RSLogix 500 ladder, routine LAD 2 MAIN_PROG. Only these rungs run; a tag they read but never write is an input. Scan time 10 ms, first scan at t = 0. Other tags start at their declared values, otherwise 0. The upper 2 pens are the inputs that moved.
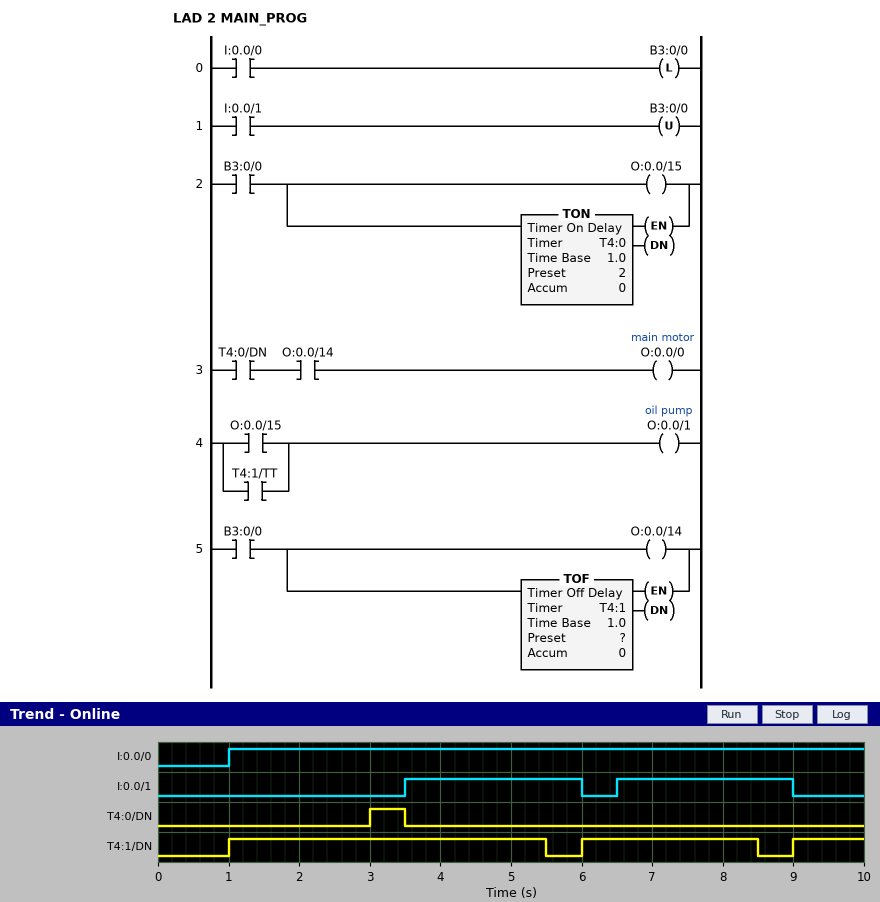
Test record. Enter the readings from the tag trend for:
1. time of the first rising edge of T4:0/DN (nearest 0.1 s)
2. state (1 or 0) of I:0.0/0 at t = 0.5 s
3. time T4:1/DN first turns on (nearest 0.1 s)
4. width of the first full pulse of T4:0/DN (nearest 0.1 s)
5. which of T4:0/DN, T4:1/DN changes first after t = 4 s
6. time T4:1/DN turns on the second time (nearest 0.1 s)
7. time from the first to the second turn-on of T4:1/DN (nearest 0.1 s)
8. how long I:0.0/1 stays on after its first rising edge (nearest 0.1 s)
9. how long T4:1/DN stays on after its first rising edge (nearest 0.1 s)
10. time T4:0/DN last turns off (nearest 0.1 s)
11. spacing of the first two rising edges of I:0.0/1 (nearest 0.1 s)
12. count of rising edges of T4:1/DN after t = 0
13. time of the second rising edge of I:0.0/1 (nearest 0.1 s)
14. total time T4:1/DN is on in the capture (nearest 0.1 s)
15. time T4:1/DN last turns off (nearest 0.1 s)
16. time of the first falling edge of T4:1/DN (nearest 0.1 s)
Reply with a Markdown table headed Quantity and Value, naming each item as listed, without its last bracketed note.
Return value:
| Quantity | Value |
|---|---|
| time of the first rising edge of T4:0/DN | 3.0 s |
| state (1 or 0) of I:0.0/0 at t = 0.5 s | 0 |
| time T4:1/DN first turns on | 1.0 s |
| width of the first full pulse of T4:0/DN | 0.5 s |
| which of T4:0/DN, T4:1/DN changes first after t = 4 s | T4:1/DN |
| time T4:1/DN turns on the second time | 6.0 s |
| time from the first to the second turn-on of T4:1/DN | 5.0 s |
| how long I:0.0/1 stays on after its first rising edge | 2.5 s |
| how long T4:1/DN stays on after its first rising edge | 4.5 s |
| time T4:0/DN last turns off | 3.5 s |
| spacing of the first two rising edges of I:0.0/1 | 3.0 s |
| count of rising edges of T4:1/DN after t = 0 | 3 |
| time of the second rising edge of I:0.0/1 | 6.5 s |
| total time T4:1/DN is on in the capture | 8.0 s |
| time T4:1/DN last turns off | 8.5 s |
| time of the first falling edge of T4:1/DN | 5.5 s |
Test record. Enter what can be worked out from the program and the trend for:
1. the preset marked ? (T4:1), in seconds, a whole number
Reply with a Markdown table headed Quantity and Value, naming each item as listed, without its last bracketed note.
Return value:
| Quantity | Value |
|---|---|
| the preset marked ? (T4:1), in seconds, a whole number | 2 s |
